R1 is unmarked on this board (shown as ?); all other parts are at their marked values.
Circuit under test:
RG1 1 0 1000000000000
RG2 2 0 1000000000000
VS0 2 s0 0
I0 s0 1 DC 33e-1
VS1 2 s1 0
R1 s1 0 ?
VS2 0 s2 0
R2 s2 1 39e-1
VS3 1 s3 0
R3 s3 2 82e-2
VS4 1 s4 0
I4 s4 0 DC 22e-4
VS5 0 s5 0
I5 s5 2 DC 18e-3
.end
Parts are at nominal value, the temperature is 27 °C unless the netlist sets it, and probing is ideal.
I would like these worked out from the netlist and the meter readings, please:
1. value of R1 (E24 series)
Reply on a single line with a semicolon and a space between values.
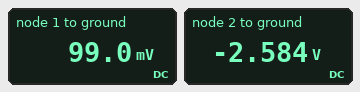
270 Ω
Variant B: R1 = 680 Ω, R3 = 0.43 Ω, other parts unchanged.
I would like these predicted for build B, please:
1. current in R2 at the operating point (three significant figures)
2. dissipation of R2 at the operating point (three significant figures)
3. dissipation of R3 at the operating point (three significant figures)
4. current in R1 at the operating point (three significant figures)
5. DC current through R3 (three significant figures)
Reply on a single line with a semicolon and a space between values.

17.8 mA; 1.23 mW; 4.63 W; 1.97 mA; 3.28 A
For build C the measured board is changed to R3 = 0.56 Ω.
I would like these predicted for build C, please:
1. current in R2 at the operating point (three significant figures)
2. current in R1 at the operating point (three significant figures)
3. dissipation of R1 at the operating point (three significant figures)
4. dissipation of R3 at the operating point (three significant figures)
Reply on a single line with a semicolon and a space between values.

22.3 mA; 6.47 mA; 11.3 mW; 6.01 W
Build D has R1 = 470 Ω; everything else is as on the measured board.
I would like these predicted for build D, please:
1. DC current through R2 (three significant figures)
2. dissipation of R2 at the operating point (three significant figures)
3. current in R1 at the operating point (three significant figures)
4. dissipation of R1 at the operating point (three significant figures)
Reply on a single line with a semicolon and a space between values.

21.3 mA; 1.78 mW; 5.54 mA; 14.4 mW
